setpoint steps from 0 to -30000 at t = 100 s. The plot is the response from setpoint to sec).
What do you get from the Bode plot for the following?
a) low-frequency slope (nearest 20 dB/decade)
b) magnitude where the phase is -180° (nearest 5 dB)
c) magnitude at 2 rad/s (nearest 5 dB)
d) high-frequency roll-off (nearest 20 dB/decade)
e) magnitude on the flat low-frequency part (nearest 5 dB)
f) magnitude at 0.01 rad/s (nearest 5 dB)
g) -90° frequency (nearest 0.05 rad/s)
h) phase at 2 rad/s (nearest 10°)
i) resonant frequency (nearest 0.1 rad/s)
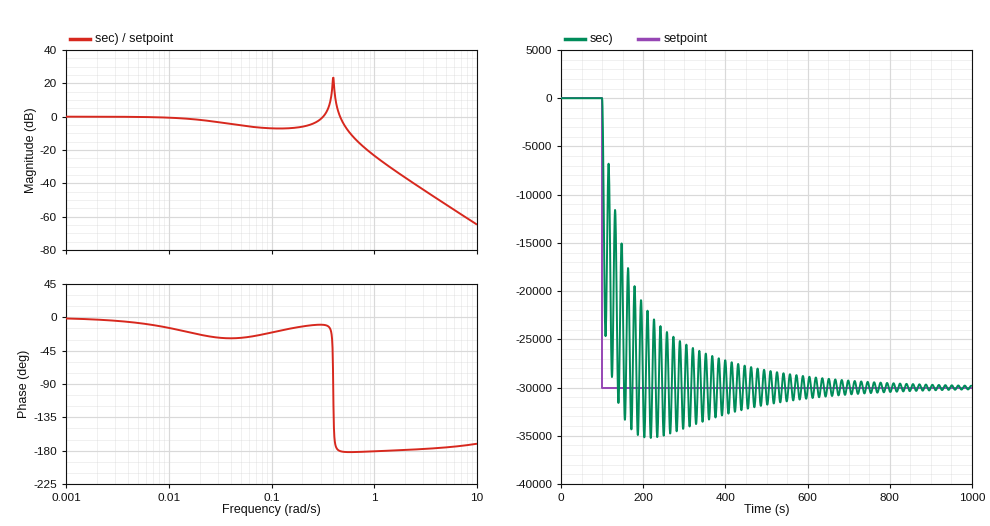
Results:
0 dB/decade
0 dB
-35 dB
-40 dB/decade
0 dB
0 dB
0.40 rad/s
-180°
0.4 rad/s
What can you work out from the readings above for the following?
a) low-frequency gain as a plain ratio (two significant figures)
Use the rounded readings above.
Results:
1.0
